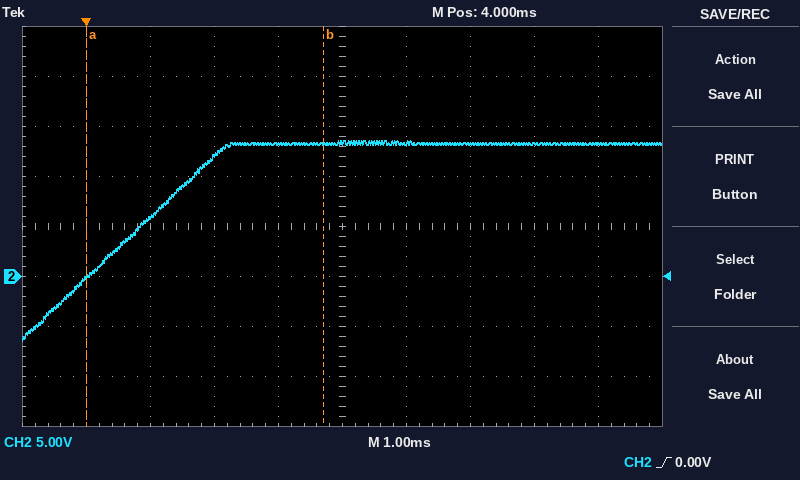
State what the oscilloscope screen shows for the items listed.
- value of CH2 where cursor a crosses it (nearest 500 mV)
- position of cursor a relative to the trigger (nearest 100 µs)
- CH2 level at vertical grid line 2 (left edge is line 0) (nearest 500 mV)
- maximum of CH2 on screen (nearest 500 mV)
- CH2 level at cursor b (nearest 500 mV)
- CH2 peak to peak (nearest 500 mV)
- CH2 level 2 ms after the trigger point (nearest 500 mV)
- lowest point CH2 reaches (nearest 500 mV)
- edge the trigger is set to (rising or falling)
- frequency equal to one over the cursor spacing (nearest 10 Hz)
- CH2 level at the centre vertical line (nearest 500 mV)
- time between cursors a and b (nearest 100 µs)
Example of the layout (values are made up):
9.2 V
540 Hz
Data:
0.0 V
0.0 ms
6.0 V
13.5 V
13.5 V
20.0 V
12.0 V
-6.5 V
rising
270 Hz
13.5 V
3.7 ms
